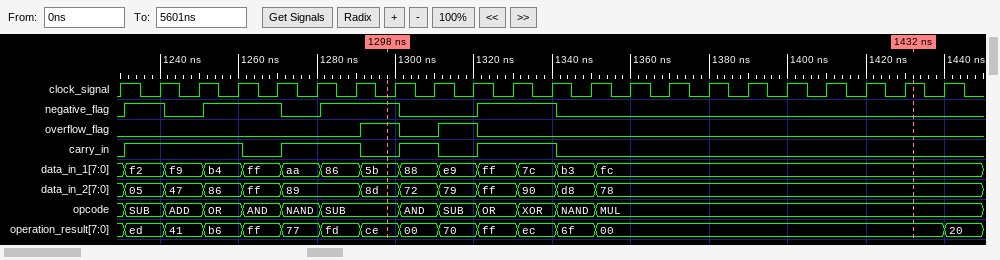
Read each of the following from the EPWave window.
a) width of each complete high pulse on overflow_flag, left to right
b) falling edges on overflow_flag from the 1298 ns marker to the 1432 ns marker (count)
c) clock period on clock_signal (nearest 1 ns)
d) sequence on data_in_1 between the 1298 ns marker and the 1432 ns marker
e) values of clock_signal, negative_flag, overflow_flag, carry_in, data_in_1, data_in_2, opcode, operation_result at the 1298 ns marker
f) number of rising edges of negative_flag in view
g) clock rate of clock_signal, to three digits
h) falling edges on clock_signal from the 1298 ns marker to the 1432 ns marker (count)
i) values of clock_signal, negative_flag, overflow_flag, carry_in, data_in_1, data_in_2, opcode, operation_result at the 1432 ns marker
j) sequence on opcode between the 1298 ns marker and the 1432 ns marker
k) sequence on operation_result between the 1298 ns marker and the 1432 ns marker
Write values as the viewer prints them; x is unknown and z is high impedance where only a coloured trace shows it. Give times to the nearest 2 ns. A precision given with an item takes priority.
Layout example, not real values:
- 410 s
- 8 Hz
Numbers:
- 10 ns, 10 ns
- 2
- 10 ns
- 5b, 88, e9, ff, 7c, b3, fc
- clock_signal=0, negative_flag=1, overflow_flag=1, carry_in=0, data_in_1=5b, data_in_2=8d, opcode=SUB, operation_result=ce
- 4
- 100 MHz
- 13
- clock_signal=1, negative_flag=0, overflow_flag=0, carry_in=0, data_in_1=fc, data_in_2=78, opcode=MUL, operation_result=00
- SUB, AND, SUB, OR, XOR, NAND, MUL
- ce, 00, 70, ff, ec, 6f, 00
